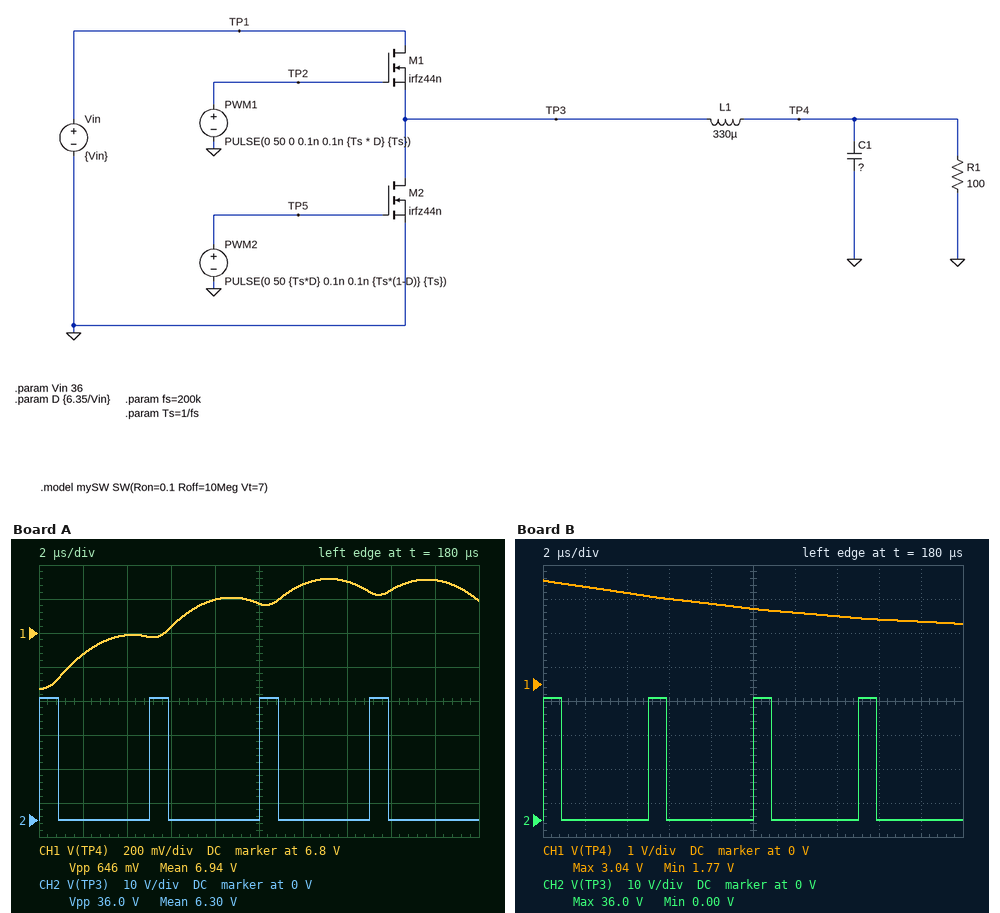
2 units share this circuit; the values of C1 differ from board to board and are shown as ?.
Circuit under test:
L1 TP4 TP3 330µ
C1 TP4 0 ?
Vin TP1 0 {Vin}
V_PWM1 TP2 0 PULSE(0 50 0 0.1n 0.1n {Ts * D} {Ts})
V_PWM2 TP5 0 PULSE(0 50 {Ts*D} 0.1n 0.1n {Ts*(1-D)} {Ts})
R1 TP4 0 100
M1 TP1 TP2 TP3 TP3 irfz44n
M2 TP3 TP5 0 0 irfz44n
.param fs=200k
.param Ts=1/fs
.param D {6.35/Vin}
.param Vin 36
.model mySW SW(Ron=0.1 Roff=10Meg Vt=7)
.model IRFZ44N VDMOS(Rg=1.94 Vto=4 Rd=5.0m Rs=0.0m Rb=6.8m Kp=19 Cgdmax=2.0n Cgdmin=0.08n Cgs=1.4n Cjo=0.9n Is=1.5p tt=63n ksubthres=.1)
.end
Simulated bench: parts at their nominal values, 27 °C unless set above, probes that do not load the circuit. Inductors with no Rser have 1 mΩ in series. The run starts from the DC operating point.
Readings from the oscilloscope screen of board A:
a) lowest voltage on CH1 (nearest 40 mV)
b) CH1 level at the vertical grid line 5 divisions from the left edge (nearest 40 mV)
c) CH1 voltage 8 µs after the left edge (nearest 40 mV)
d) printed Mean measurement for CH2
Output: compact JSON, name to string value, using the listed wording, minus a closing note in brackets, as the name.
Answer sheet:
{"lowest voltage on CH1": "6.48 V", "CH1 level at the vertical grid line 5 divisions from the left edge": "6.96 V", "CH1 voltage 8 µs after the left edge": "7.00 V", "printed Mean measurement for CH2": "6.30 V"}
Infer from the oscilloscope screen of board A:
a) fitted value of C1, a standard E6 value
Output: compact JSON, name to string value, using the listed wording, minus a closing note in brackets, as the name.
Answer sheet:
{"fitted value of C1, a standard E6 value": "470 nF"}
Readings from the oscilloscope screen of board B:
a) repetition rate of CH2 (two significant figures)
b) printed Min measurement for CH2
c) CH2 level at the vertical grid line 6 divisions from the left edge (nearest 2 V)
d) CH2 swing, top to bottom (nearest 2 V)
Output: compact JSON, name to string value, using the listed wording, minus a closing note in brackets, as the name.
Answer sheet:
{"repetition rate of CH2": "200 kHz", "printed Min measurement for CH2": "0.00 V", "CH2 level at the vertical grid line 6 divisions from the left edge": "0 V", "CH2 swing, top to bottom": "36 V"}
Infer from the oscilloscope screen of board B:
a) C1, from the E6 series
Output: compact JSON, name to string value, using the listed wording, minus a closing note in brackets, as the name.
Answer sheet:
{"C1, from the E6 series": "3.3 µF"}
